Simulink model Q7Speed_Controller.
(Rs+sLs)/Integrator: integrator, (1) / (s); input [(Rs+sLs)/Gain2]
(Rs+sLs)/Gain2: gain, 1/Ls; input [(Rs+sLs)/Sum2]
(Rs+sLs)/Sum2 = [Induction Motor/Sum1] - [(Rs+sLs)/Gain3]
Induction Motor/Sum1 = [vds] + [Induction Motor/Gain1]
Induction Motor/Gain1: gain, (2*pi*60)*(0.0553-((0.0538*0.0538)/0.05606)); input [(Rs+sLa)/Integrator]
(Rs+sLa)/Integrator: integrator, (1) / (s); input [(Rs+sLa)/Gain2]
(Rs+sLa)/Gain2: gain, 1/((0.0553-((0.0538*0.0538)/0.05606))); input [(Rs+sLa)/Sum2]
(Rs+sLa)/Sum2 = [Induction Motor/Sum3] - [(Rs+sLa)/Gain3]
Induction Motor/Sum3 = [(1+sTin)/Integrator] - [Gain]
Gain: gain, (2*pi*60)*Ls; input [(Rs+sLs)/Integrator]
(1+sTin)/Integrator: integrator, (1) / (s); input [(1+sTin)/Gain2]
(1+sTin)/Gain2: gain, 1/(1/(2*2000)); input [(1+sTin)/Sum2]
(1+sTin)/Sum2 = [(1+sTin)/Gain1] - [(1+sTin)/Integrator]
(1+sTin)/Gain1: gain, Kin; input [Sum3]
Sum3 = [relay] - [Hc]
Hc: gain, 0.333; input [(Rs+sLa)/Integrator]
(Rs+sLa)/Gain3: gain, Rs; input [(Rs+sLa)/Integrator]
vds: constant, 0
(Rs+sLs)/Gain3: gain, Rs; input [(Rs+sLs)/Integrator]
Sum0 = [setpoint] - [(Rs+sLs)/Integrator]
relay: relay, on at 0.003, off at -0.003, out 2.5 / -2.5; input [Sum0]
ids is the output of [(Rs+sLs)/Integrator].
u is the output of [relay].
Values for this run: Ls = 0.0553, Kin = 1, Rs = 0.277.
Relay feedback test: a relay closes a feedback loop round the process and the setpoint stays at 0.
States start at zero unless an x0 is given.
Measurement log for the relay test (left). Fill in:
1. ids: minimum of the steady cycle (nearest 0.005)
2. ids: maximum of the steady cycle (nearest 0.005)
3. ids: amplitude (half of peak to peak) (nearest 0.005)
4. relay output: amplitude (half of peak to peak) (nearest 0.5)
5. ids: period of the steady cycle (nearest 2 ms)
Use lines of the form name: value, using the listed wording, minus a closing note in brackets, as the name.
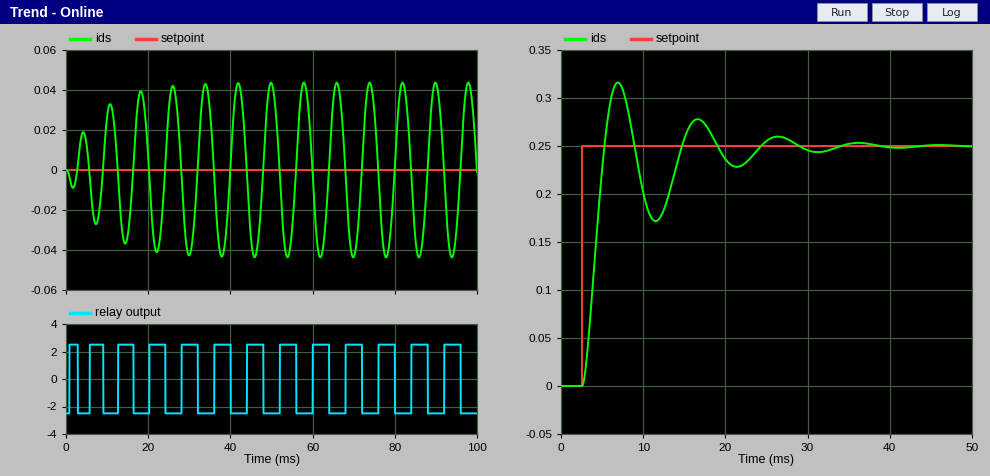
ids: minimum of the steady cycle: -0.045
ids: maximum of the steady cycle: 0.045
ids: amplitude (half of peak to peak): 0.045
relay output: amplitude (half of peak to peak): 2.5
ids: period of the steady cycle: 8 ms
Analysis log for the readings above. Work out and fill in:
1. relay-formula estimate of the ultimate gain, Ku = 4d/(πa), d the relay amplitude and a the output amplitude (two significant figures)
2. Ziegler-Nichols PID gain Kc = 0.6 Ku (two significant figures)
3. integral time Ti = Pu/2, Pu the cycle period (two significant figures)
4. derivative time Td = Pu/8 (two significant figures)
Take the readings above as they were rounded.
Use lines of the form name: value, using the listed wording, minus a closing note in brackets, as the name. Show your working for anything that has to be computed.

relay-formula estimate of the ultimate gain, Ku = 4d/(πa), d the relay amplitude and a the output amplitude: 4 × 2.5 / (π × 0.045) = 71
Ziegler-Nichols PID gain Kc = 0.6 Ku: 0.6 × 71 = 43
integral time Ti = Pu/2, Pu the cycle period: 8 / 2 = 4.0 ms
derivative time Td = Pu/8: 8 / 8 = 1.0 ms
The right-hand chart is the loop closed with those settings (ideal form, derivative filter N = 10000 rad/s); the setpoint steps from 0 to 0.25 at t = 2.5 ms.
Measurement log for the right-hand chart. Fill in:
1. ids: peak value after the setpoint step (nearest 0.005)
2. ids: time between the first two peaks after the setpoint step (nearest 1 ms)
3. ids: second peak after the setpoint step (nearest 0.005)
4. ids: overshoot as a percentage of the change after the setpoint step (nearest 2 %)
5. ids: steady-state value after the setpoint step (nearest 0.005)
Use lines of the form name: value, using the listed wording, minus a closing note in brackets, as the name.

ids: peak value after the setpoint step: 0.315
ids: time between the first two peaks after the setpoint step: 10 ms
ids: second peak after the setpoint step: 0.280
ids: overshoot as a percentage of the change after the setpoint step: 26 %
ids: steady-state value after the setpoint step: 0.250
